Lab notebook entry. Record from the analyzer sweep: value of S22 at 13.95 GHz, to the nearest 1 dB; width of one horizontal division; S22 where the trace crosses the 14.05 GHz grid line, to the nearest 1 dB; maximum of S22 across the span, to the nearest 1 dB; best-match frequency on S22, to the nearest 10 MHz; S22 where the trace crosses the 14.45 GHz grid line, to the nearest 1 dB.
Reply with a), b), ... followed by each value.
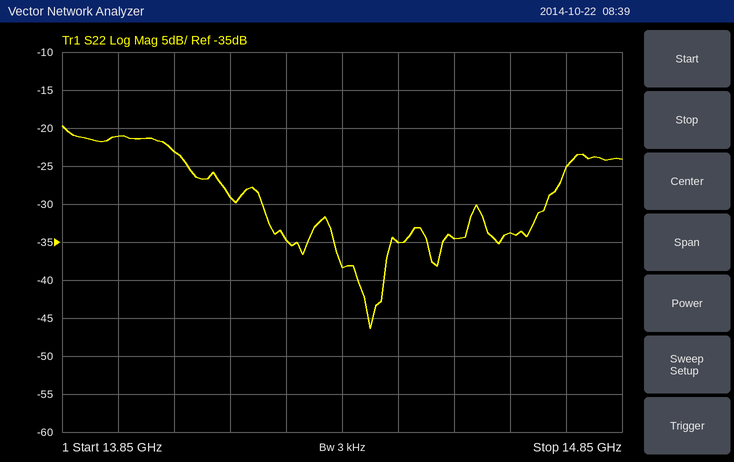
a) -21 dB
b) 100 MHz
c) -23 dB
d) -20 dB
e) 14.40 GHz
f) -35 dB
